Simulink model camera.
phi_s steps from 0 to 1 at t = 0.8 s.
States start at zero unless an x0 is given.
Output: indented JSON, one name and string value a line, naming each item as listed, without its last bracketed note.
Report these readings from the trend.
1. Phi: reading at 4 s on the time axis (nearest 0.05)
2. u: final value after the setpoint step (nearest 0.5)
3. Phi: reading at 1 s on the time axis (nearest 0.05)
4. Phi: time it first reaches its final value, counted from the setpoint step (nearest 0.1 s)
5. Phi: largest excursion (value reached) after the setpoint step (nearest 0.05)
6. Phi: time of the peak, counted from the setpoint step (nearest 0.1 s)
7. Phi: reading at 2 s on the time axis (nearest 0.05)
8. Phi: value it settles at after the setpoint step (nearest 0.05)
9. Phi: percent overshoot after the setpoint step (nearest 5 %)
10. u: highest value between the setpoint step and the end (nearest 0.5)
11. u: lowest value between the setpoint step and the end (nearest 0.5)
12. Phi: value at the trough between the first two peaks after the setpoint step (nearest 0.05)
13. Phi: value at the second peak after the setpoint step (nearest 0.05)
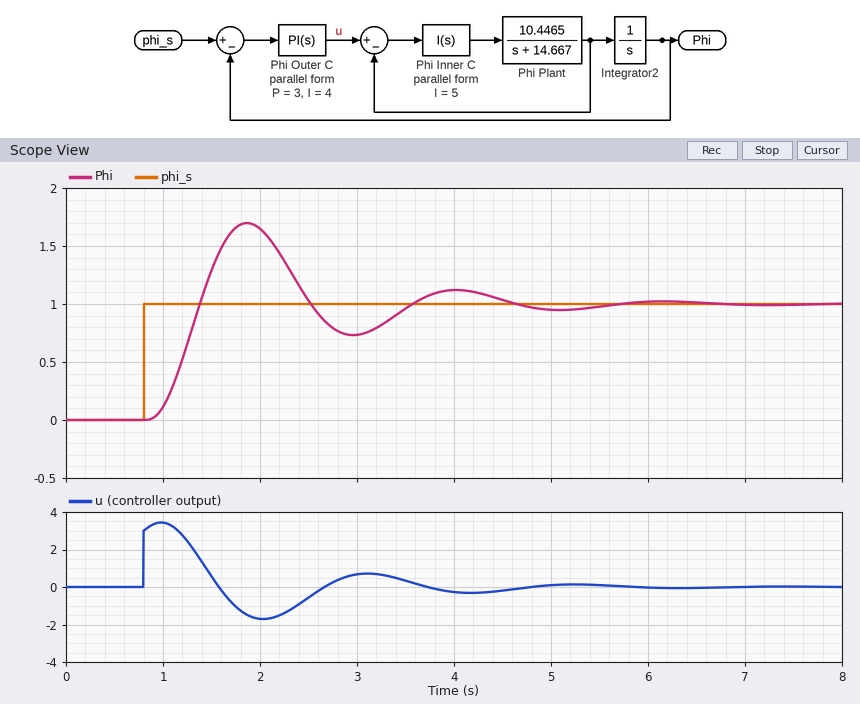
{
  "Phi: reading at 4 s on the time axis": "1.10",
  "u: final value after the setpoint step": "0.0",
  "Phi: reading at 1 s on the time axis": "0.10",
  "Phi: time it first reaches its final value, counted from the setpoint step": "0.6 s",
  "Phi: largest excursion (value reached) after the setpoint step": "1.70",
  "Phi: time of the peak, counted from the setpoint step": "1.1 s",
  "Phi: reading at 2 s on the time axis": "1.65",
  "Phi: value it settles at after the setpoint step": "1.00",
  "Phi: percent overshoot after the setpoint step": "70 %",
  "u: highest value between the setpoint step and the end": "3.5",
  "u: lowest value between the setpoint step and the end": "-1.5",
  "Phi: value at the trough between the first two peaks after the setpoint step": "0.75",
  "Phi: value at the second peak after the setpoint step": "1.10"
}
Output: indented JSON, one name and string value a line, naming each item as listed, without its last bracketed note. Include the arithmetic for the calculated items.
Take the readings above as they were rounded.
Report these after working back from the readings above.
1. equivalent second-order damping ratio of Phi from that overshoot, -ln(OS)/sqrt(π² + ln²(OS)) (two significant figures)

{
  "equivalent second-order damping ratio of Phi from that overshoot, -ln(OS)/sqrt(π² + ln²(OS))": "ln(0.7) = -0.357; 0.357 / sqrt(9.870 + 0.127) = 0.11"
}
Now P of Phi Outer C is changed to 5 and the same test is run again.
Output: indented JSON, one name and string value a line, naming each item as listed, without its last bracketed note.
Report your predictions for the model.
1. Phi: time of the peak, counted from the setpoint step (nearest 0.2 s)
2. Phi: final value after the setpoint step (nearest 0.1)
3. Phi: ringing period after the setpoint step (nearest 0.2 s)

{
  "Phi: time of the peak, counted from the setpoint step": "0.8 s",
  "Phi: final value after the setpoint step": "1.0",
  "Phi: ringing period after the setpoint step": "1.4 s"
}
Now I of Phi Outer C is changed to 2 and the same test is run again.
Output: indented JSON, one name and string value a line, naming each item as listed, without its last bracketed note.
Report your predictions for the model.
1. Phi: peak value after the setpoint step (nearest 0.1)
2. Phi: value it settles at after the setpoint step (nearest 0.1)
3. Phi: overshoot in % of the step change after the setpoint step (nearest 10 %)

{
  "Phi: peak value after the setpoint step": "1.5",
  "Phi: value it settles at after the setpoint step": "1.0",
  "Phi: overshoot in % of the step change after the setpoint step": "50 %"
}
